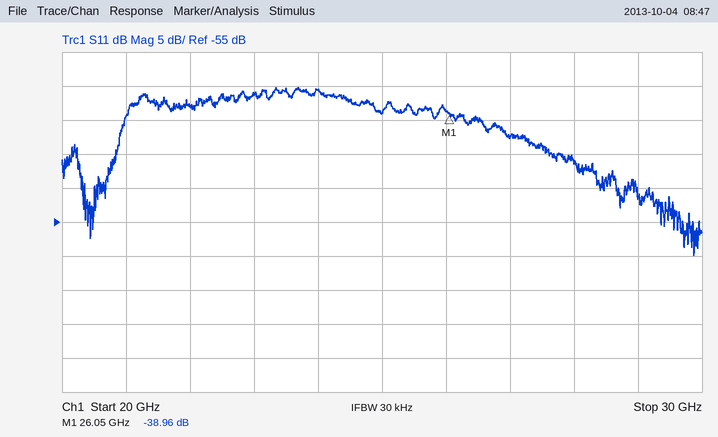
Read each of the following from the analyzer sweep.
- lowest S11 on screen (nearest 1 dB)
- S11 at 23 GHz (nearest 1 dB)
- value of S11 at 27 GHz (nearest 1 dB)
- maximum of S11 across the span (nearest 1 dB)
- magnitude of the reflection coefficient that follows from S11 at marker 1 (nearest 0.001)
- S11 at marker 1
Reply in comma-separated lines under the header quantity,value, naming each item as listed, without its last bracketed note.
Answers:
quantity,value
lowest S11 on screen,-60 dB
S11 at 23 GHz,-36 dB
value of S11 at 27 GHz,-42 dB
maximum of S11 across the span,-35 dB
magnitude of the reflection coefficient that follows from S11 at marker 1,0.011
S11 at marker 1,-38.96 dB
